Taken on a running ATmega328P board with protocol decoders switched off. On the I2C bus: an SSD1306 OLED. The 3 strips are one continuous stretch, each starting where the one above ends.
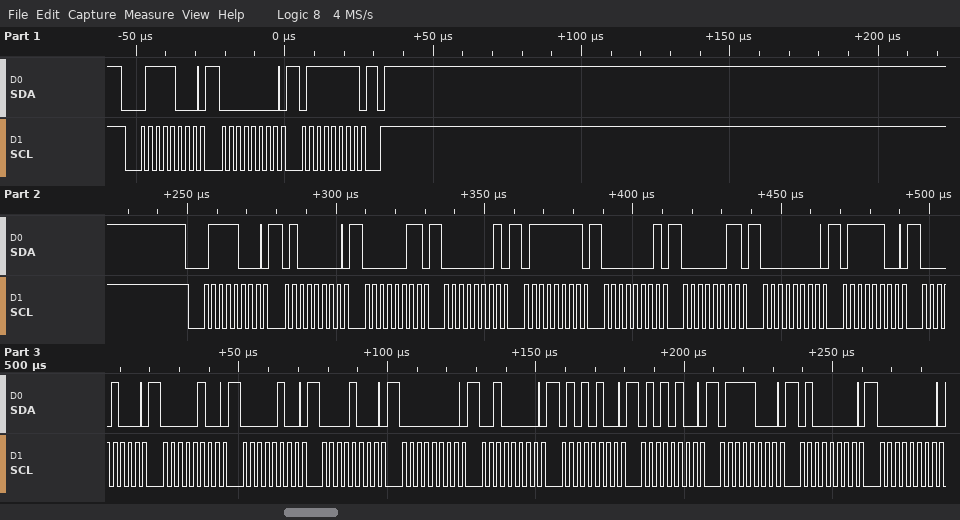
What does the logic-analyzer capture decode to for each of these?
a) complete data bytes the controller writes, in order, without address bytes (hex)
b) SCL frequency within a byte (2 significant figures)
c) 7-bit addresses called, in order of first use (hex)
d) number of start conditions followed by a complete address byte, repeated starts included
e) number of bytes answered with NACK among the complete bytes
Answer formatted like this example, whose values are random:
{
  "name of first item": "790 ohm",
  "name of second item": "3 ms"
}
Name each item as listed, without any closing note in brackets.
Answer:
{
  "complete data bytes the controller writes, in order, without address bytes": "00 7F 40 03 01 7F 01 03 00 7C 08 04 04 08 00 20 54 54 78 40 00",
  "SCL frequency within a byte": "400 kHz",
  "7-bit addresses called, in order of first use": "0x3C",
  "number of start conditions followed by a complete address byte, repeated starts included": "2",
  "number of bytes answered with NACK among the complete bytes": "0"
}
